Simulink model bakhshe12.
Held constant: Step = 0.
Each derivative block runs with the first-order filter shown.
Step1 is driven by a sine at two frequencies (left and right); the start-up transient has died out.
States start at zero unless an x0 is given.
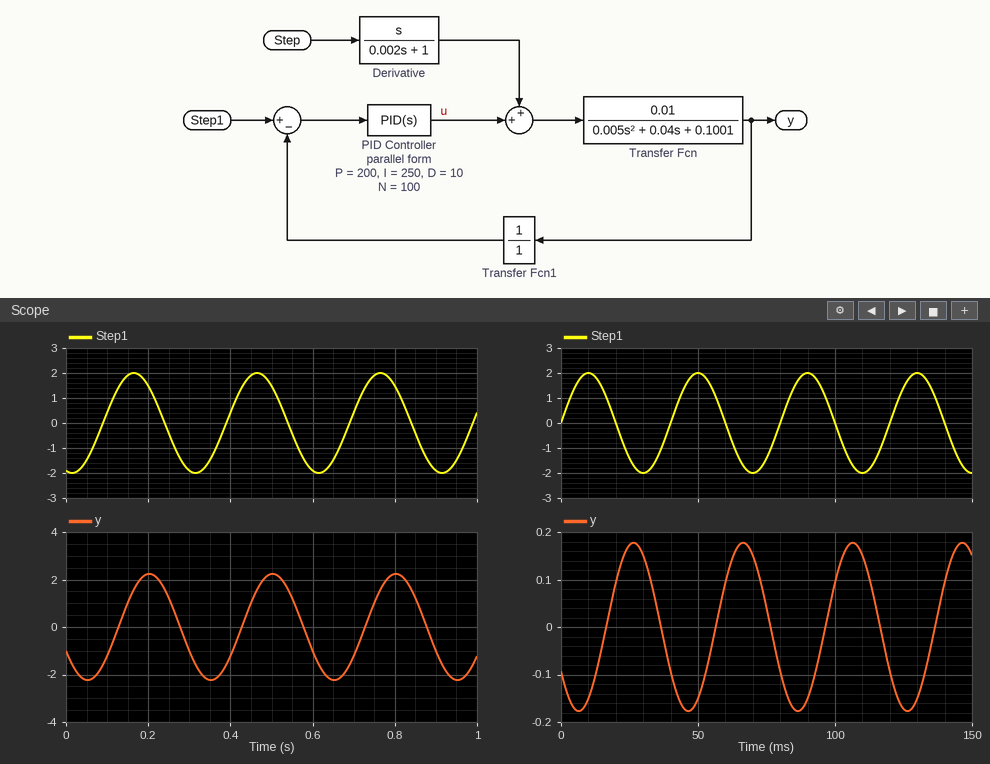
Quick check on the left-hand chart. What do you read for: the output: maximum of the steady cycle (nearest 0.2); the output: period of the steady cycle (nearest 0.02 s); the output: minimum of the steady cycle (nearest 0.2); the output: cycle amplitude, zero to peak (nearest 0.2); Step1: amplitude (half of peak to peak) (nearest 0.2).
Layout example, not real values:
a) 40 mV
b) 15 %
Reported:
a) 2.2
b) 0.30 s
c) -2.2
d) 2.2
e) 2.0
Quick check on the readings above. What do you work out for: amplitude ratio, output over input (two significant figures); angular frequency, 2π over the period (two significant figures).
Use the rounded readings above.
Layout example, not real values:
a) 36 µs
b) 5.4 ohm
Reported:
a) 1.1
b) 21 rad/s
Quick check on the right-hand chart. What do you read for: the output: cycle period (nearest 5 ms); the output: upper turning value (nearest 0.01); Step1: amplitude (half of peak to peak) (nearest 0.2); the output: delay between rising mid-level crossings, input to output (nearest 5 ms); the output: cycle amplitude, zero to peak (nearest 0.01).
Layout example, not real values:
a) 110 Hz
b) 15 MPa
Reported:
a) 40 ms
b) 0.18
c) 2.0
d) 15 ms
e) 0.18
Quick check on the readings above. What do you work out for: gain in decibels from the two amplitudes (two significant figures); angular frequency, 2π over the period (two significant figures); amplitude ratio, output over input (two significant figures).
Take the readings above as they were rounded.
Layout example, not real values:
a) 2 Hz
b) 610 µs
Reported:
a) -21 dB
b) 0.16 rad/ms
c) 0.090
